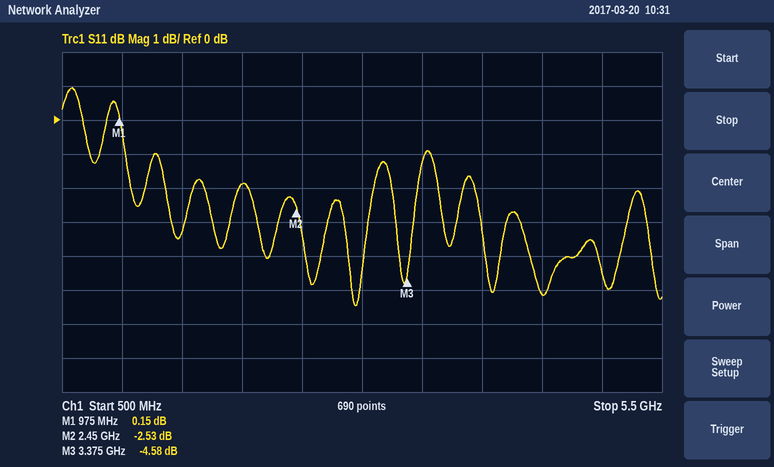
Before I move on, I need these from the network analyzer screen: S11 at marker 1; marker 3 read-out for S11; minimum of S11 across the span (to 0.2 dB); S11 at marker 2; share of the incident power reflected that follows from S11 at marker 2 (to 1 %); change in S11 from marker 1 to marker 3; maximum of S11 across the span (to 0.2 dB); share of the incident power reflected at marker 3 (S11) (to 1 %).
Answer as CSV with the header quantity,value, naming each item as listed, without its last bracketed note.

quantity,value
S11 at marker 1,0.15 dB
marker 3 read-out for S11,-4.58 dB
minimum of S11 across the span,-5.4 dB
S11 at marker 2,-2.53 dB
share of the incident power reflected that follows from S11 at marker 2,56 %
change in S11 from marker 1 to marker 3,-4.73 dB
maximum of S11 across the span,1.0 dB
share of the incident power reflected at marker 3 (S11),35 %
